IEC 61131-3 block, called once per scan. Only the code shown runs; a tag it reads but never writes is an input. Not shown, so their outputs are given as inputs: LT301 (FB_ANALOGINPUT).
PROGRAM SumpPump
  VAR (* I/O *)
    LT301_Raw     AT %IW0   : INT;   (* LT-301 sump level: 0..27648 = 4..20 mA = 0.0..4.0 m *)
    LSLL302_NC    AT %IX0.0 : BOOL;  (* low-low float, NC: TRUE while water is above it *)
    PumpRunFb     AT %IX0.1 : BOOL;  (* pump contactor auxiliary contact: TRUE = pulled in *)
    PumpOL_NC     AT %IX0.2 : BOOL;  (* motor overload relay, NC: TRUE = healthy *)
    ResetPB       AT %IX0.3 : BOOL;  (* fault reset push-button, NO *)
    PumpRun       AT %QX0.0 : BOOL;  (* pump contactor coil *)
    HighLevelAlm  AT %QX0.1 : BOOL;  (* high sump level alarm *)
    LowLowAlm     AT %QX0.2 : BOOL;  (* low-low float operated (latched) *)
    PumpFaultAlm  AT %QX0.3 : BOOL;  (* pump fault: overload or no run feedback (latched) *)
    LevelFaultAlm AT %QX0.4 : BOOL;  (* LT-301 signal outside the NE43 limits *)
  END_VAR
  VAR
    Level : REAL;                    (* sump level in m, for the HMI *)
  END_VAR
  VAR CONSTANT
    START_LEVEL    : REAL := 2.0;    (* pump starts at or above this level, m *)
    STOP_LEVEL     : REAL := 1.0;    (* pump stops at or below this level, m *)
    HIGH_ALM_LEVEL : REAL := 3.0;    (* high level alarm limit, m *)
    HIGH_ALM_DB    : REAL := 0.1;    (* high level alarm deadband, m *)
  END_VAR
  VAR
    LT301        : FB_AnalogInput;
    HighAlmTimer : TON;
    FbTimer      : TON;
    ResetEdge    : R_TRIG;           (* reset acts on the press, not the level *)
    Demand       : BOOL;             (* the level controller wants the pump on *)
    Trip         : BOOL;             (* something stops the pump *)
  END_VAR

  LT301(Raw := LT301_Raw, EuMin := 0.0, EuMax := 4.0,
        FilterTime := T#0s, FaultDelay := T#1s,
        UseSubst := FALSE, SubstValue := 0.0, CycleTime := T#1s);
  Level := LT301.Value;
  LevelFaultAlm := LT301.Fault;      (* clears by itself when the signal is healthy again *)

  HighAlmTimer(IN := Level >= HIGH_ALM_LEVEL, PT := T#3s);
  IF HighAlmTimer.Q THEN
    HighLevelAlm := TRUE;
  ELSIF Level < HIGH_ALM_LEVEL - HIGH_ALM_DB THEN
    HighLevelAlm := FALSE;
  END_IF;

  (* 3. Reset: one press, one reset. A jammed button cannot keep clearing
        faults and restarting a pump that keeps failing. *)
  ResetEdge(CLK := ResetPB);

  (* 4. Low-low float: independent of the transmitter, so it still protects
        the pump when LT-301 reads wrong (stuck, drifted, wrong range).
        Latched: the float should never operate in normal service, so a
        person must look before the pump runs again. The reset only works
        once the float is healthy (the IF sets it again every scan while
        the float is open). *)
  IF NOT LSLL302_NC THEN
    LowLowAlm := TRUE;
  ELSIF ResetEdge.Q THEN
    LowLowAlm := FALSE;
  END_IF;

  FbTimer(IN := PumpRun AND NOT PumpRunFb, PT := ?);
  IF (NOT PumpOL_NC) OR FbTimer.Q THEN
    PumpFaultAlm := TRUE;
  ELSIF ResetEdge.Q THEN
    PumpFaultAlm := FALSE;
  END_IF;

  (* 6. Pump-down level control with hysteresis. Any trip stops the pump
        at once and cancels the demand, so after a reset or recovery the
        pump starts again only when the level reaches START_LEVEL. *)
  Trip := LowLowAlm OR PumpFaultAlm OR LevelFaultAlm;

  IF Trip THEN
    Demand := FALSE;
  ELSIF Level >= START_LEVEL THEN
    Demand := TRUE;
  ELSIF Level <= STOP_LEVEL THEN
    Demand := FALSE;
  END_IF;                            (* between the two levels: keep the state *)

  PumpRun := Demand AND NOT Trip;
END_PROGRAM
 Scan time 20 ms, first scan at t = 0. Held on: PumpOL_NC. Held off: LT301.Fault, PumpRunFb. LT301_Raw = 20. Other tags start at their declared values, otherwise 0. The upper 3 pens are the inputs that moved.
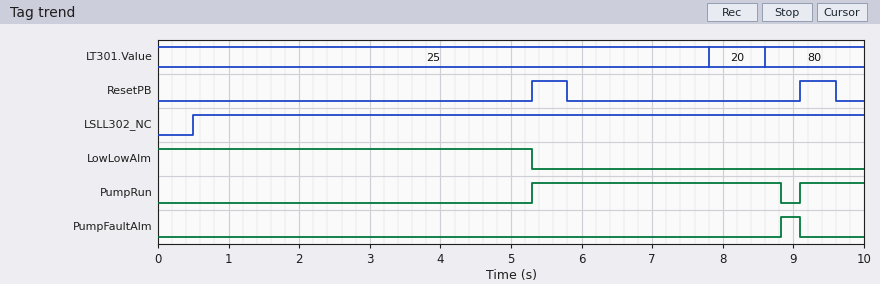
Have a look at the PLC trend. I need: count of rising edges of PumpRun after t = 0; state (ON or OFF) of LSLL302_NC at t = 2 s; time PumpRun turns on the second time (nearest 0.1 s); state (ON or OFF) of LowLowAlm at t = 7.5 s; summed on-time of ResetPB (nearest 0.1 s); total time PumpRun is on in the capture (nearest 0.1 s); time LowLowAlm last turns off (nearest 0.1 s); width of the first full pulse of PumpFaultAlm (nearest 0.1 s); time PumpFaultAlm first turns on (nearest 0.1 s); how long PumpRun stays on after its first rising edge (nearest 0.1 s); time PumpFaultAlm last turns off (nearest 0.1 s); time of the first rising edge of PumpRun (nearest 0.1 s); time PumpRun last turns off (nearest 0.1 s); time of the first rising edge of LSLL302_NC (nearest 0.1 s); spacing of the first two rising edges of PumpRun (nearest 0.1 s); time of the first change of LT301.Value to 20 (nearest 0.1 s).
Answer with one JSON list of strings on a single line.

["2", "ON", "9.1 s", "OFF", "1.0 s", "4.4 s", "5.3 s", "0.3 s", "8.8 s", "3.5 s", "9.1 s", "5.3 s", "8.8 s", "0.5 s", "3.8 s", "7.8 s"]
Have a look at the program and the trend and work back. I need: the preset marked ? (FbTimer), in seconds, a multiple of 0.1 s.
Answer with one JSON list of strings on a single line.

["3.5 s"]
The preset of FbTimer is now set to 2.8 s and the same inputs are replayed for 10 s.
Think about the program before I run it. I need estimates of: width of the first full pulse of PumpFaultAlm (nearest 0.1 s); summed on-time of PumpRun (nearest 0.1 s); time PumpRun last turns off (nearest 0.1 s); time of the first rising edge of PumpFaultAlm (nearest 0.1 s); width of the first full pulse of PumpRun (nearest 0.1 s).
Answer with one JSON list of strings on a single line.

["1.0 s", "3.7 s", "8.1 s", "8.1 s", "2.8 s"]
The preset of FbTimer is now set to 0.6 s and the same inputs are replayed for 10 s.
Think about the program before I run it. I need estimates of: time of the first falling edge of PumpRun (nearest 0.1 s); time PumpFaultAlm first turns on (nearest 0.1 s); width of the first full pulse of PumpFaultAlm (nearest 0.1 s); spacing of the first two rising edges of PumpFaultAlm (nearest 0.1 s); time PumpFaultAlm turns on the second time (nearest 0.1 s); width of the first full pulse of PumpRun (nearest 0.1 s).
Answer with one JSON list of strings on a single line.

["5.9 s", "5.9 s", "3.2 s", "3.8 s", "9.7 s", "0.6 s"]
